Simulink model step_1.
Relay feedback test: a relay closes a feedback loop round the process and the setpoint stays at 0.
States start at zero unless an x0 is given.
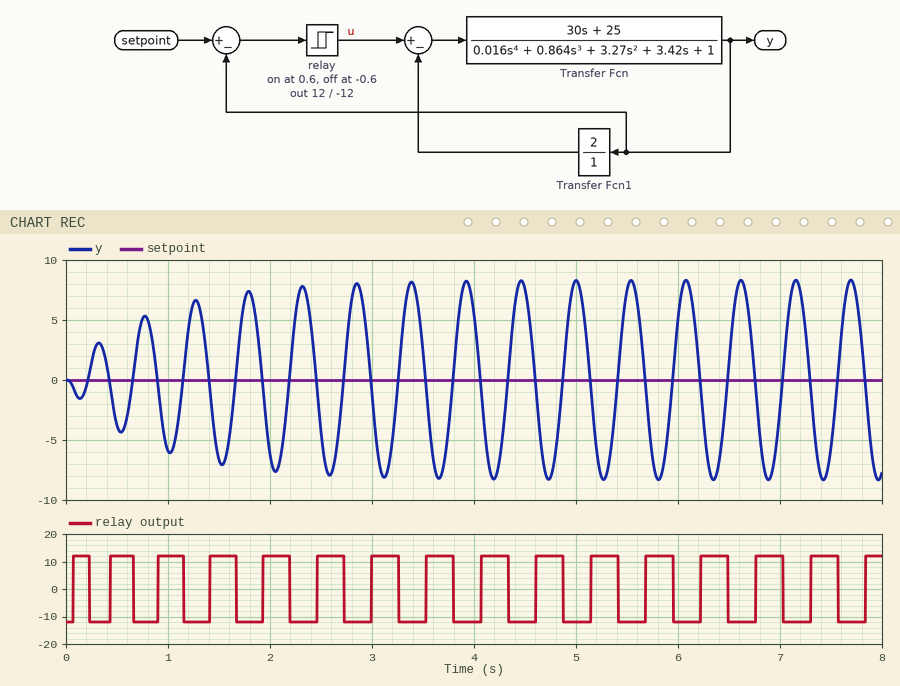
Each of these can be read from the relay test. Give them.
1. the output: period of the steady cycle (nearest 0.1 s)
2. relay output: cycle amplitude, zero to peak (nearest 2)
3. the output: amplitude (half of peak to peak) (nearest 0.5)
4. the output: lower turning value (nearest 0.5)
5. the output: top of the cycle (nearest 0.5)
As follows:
0.5 s
12
8.5
-8.5
8.5
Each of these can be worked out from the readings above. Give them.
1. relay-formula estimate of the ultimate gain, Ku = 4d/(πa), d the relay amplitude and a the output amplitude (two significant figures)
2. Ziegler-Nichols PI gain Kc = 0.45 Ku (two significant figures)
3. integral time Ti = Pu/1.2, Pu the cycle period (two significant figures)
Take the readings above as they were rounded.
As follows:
1.8
0.81
0.42 s
